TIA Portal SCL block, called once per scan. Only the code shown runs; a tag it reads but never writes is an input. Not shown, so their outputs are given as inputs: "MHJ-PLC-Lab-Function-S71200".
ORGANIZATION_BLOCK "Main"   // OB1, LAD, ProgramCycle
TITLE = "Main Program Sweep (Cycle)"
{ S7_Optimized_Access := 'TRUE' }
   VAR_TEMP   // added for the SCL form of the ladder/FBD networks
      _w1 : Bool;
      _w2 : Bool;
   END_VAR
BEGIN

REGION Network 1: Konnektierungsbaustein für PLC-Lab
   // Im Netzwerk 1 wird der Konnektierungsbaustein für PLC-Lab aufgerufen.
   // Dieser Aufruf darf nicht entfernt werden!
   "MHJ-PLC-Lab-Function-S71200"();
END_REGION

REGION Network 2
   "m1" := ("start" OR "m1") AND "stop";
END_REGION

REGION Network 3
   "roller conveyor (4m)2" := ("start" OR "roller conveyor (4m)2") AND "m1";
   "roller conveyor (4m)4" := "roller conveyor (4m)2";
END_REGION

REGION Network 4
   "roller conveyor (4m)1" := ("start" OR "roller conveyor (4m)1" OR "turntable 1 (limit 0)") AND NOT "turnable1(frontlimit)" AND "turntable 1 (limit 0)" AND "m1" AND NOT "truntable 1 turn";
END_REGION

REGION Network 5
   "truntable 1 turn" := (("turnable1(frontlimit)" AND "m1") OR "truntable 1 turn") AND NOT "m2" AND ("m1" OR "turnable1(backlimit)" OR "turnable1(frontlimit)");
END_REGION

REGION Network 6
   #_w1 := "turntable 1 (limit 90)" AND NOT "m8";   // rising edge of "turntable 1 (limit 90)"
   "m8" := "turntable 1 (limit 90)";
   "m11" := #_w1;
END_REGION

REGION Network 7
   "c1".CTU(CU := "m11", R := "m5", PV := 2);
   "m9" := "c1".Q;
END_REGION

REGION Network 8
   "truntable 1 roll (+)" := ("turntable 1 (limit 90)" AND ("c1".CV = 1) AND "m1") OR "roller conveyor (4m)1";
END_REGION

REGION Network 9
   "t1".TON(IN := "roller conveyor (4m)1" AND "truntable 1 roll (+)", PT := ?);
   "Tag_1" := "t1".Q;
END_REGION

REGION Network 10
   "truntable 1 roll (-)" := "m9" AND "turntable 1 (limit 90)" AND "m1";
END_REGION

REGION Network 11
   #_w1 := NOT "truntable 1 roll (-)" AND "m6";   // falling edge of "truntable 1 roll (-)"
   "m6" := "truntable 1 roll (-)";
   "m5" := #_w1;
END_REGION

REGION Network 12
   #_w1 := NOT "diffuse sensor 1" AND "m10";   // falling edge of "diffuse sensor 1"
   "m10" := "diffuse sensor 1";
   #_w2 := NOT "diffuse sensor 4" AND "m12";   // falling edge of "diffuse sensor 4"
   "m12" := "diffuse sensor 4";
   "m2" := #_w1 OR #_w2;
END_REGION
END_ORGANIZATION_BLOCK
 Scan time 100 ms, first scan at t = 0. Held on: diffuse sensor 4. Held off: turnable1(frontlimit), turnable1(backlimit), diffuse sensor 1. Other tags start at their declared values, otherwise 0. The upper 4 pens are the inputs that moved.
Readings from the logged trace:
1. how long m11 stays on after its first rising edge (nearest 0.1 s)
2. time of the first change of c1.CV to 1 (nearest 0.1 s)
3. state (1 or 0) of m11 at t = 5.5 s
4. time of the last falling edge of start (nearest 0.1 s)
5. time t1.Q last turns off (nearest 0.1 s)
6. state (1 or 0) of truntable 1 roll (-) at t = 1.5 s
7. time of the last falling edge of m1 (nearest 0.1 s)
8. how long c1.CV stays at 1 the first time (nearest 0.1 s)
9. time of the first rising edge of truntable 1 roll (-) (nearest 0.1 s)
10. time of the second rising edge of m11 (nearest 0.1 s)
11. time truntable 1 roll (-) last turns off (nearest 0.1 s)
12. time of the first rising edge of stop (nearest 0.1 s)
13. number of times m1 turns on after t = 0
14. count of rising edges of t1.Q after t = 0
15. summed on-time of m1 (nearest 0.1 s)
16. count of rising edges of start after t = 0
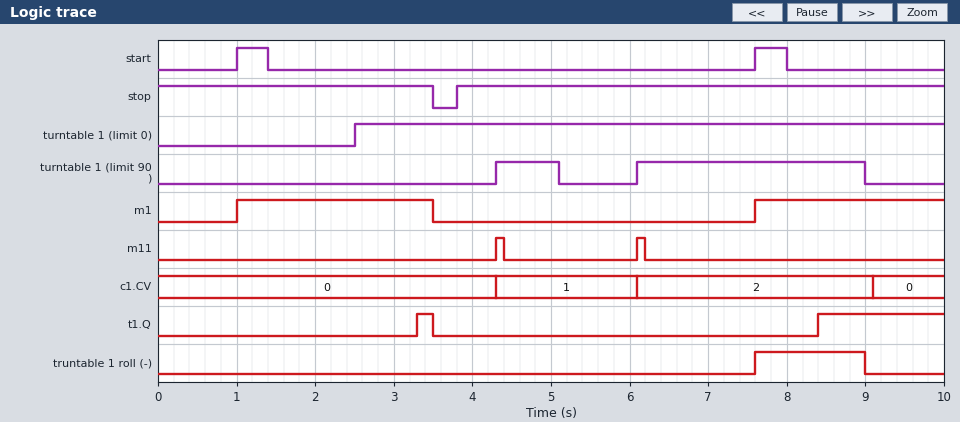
0.1 s
4.3 s
0
8.0 s
3.5 s
0
3.5 s
1.8 s
7.6 s
6.1 s
9.0 s
3.8 s
2
2
4.9 s
2
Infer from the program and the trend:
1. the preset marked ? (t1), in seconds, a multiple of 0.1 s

0.8 s
